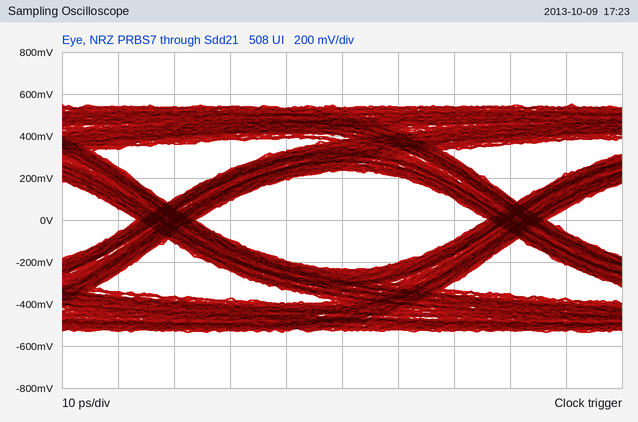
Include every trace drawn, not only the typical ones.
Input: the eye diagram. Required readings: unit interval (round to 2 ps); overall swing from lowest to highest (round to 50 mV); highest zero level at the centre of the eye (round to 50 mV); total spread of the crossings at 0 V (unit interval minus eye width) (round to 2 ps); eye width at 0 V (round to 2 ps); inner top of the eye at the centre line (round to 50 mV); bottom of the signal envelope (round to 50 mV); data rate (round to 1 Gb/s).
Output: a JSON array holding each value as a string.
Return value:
["62 ps", "1.10 V", "-250 mV", "10 ps", "52 ps", "250 mV", "-550 mV", "16 Gb/s"]
